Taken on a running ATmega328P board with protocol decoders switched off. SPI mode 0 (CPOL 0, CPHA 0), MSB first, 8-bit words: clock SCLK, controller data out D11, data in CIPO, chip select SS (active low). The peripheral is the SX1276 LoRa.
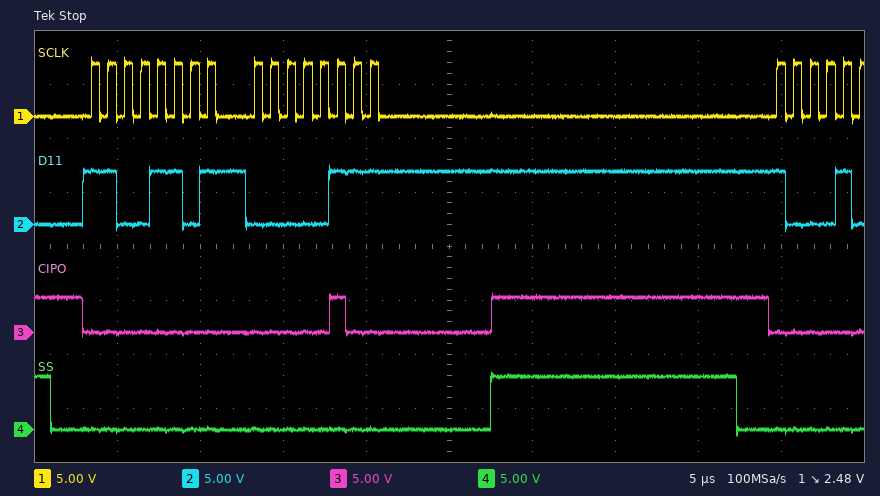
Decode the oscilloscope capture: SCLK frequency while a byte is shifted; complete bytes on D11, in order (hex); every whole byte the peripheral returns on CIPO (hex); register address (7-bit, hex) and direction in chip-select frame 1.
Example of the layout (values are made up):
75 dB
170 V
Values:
1 MHz
0xCD 0x07
0x00 0x04
0x4D write
